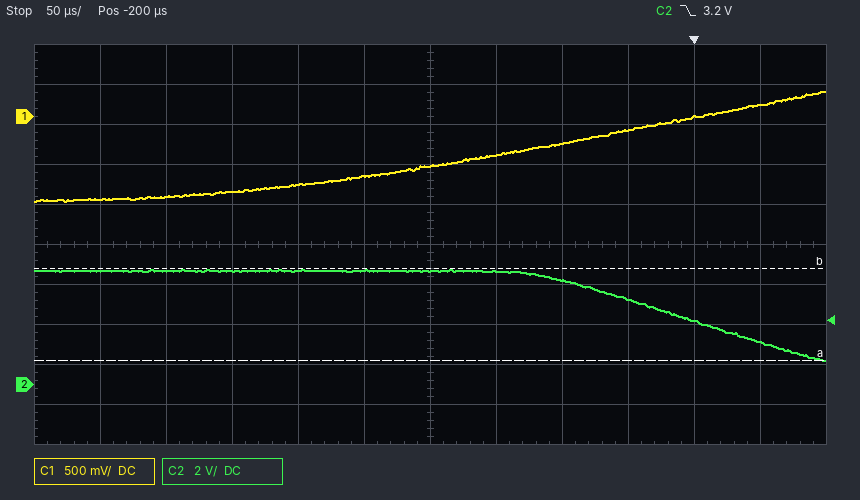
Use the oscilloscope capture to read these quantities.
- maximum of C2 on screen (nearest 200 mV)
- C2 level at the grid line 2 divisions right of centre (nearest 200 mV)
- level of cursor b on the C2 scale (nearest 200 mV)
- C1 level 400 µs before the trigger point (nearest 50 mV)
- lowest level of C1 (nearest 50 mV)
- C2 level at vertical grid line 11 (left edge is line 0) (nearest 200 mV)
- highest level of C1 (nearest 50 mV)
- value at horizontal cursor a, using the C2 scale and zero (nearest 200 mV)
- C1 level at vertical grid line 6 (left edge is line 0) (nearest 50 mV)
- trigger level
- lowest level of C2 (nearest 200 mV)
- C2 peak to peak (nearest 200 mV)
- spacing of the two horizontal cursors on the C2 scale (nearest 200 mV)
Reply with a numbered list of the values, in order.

1. 5.8 V
2. 5.2 V
3. 5.8 V
4. -1.00 V
5. -1.05 V
6. 2.2 V
7. 300 mV
8. 1.2 V
9. -600 mV
10. 3.2 V
11. 1.2 V
12. 4.6 V
13. 4.6 V
